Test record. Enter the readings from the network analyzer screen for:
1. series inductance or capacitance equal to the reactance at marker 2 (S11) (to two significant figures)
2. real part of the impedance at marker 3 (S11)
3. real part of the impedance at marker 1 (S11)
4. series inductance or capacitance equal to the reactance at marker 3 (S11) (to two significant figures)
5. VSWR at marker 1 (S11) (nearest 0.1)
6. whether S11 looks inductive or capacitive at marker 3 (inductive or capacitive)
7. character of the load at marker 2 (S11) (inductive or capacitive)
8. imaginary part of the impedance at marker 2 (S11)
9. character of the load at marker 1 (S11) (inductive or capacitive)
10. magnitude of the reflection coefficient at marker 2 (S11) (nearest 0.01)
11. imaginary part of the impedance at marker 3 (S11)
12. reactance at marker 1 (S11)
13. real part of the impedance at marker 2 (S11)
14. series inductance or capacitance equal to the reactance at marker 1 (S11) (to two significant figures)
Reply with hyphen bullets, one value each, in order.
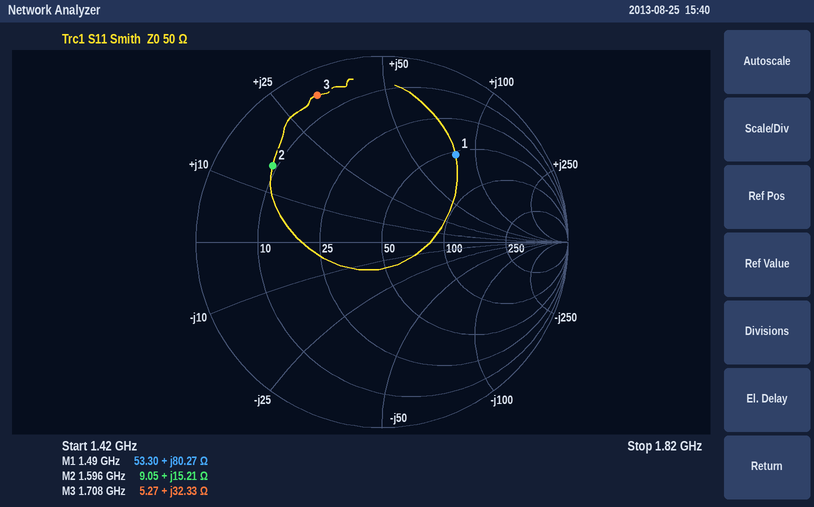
- 1.5 nH
- 5.27 Ω
- 53.30 Ω
- 3.0 nH
- 4.2
- inductive
- inductive
- +15.21 Ω
- inductive
- 0.72
- +32.33 Ω
- +80.27 Ω
- 9.05 Ω
- 8.6 nH
